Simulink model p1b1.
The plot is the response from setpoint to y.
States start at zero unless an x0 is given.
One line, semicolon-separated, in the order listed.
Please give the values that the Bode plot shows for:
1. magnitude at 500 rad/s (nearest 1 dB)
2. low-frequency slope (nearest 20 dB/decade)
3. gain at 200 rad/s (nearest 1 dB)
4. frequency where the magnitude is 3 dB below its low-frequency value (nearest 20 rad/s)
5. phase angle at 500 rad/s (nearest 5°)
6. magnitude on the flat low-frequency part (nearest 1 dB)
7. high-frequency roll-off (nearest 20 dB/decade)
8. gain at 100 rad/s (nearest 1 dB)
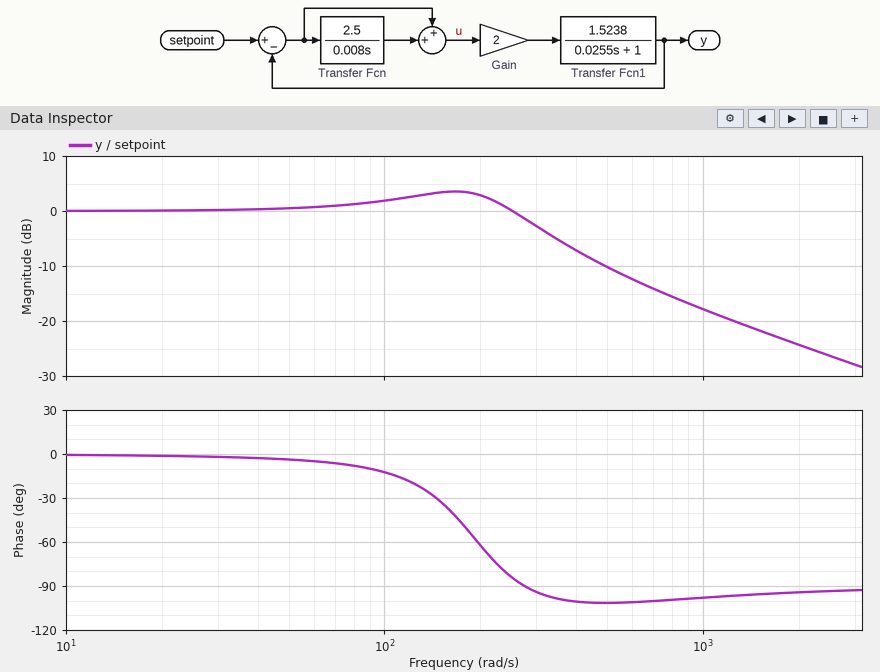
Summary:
-10 dB; 0 dB/decade; 3 dB; 300 rad/s; -100°; 0 dB; -20 dB/decade; 2 dB
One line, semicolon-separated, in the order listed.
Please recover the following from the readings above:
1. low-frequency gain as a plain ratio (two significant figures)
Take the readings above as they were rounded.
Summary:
1.0
